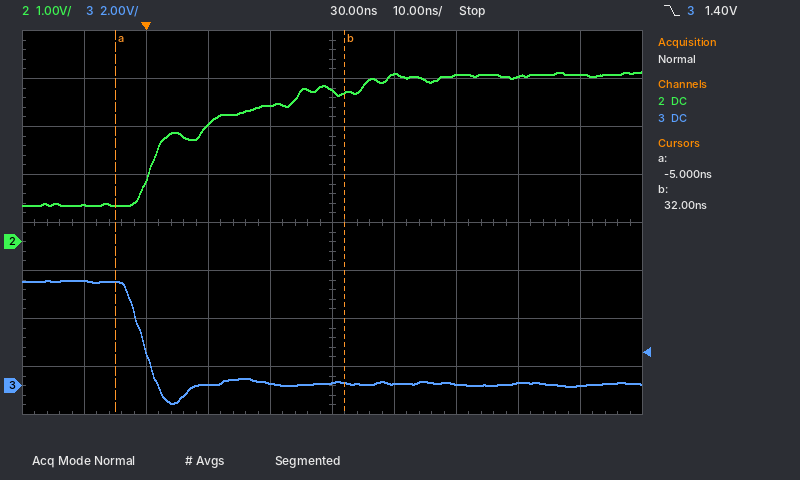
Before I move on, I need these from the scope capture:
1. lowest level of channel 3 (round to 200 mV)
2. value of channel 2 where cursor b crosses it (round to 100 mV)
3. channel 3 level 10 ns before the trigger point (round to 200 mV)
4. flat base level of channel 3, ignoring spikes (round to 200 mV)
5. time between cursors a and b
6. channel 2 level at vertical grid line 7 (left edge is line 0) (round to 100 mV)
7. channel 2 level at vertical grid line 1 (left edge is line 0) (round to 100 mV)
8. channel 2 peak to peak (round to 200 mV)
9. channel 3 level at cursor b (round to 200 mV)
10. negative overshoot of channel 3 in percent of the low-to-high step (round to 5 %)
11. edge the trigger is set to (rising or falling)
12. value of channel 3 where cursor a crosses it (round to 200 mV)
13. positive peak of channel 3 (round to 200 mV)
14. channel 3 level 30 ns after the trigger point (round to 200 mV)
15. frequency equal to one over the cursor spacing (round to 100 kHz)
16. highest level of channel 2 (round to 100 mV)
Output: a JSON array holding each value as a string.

["-800 mV", "3.1 V", "4.4 V", "0.0 V", "37 ns", "3.5 V", "800 mV", "2.8 V", "200 mV", "20 %", "falling", "4.4 V", "4.4 V", "200 mV", "27.0 MHz", "3.5 V"]
